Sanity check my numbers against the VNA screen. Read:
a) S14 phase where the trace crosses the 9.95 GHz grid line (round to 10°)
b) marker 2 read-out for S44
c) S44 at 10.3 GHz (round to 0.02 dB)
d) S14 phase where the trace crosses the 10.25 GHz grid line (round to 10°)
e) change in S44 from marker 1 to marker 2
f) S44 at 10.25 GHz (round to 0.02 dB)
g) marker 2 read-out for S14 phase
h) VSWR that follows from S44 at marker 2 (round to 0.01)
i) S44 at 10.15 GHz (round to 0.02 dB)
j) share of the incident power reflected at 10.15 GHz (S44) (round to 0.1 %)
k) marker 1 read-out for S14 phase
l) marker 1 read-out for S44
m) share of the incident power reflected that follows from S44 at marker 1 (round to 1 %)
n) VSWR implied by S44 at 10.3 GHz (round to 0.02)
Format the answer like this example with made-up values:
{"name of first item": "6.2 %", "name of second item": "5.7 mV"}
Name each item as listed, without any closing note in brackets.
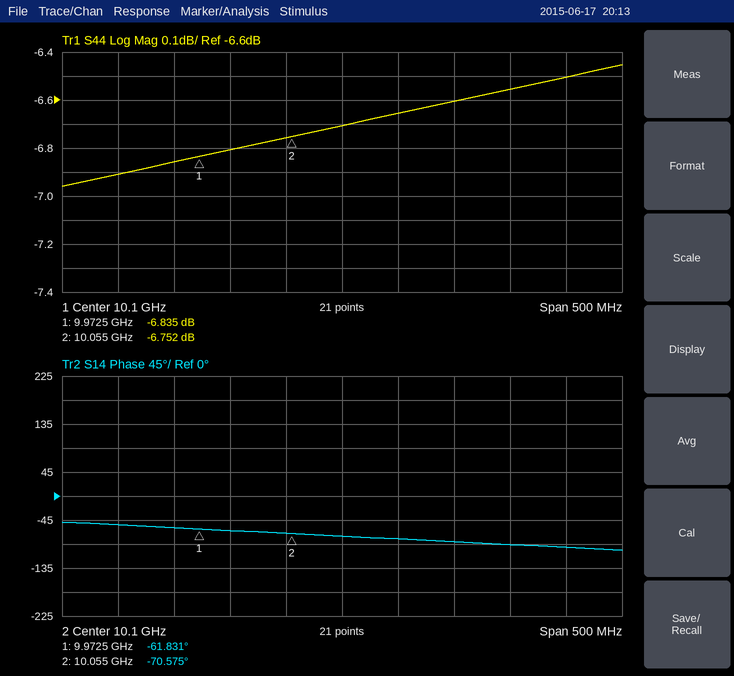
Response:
{"S14 phase where the trace crosses the 9.95 GHz grid line": "-60°", "marker 2 read-out for S44": "-6.752 dB", "S44 at 10.3 GHz": "-6.50 dB", "S14 phase where the trace crosses the 10.25 GHz grid line": "-90°", "change in S44 from marker 1 to marker 2": "0.083 dB", "S44 at 10.25 GHz": "-6.56 dB", "marker 2 read-out for S14 phase": "-70.575°", "VSWR that follows from S44 at marker 2": "2.70", "S44 at 10.15 GHz": "-6.66 dB", "share of the incident power reflected at 10.15 GHz (S44)": "21.6 %", "marker 1 read-out for S14 phase": "-61.831°", "marker 1 read-out for S44": "-6.835 dB", "share of the incident power reflected that follows from S44 at marker 1": "21 %", "VSWR implied by S44 at 10.3 GHz": "2.80"}
